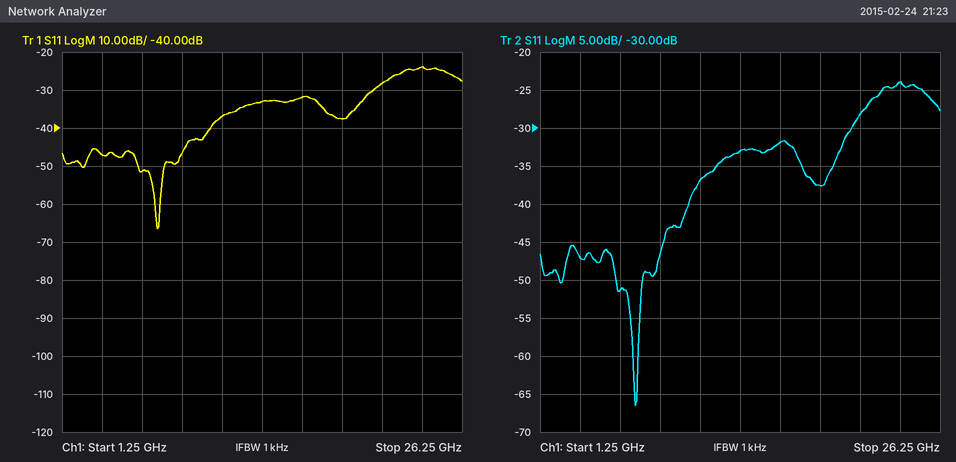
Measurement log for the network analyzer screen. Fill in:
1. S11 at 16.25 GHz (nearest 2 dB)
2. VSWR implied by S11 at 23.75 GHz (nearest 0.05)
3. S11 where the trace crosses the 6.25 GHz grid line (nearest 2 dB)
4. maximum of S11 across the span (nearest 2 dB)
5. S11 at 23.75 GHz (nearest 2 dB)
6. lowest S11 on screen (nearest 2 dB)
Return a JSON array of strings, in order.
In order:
["-32 dB", "1.15", "-52 dB", "-24 dB", "-24 dB", "-66 dB"]
